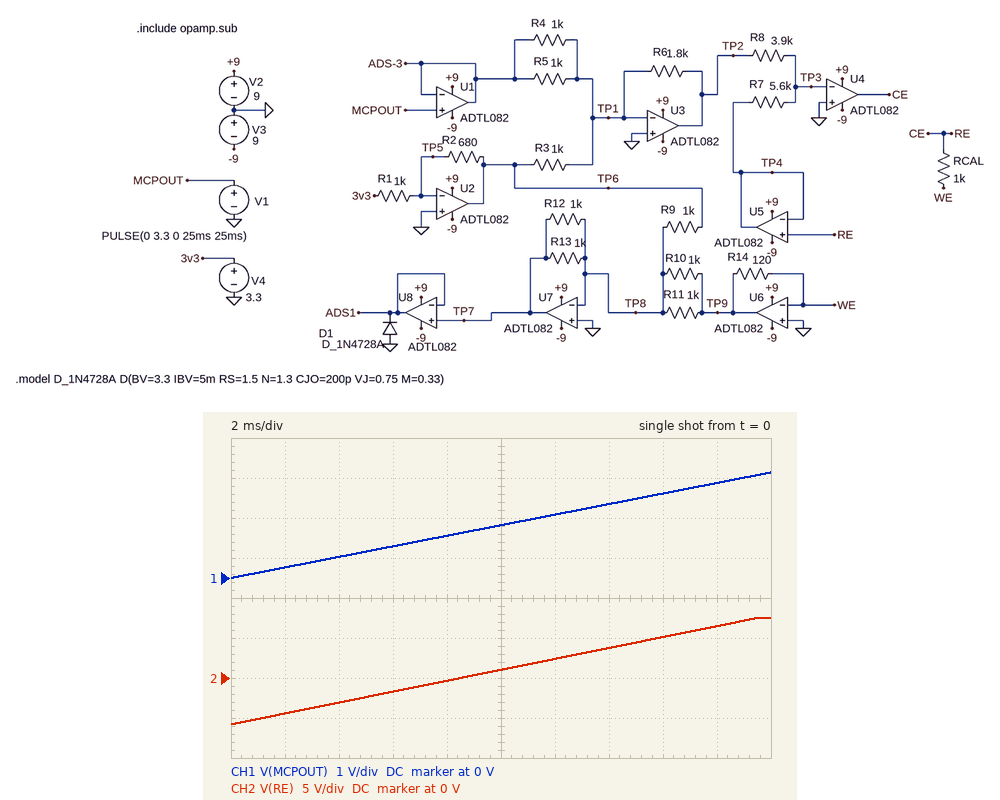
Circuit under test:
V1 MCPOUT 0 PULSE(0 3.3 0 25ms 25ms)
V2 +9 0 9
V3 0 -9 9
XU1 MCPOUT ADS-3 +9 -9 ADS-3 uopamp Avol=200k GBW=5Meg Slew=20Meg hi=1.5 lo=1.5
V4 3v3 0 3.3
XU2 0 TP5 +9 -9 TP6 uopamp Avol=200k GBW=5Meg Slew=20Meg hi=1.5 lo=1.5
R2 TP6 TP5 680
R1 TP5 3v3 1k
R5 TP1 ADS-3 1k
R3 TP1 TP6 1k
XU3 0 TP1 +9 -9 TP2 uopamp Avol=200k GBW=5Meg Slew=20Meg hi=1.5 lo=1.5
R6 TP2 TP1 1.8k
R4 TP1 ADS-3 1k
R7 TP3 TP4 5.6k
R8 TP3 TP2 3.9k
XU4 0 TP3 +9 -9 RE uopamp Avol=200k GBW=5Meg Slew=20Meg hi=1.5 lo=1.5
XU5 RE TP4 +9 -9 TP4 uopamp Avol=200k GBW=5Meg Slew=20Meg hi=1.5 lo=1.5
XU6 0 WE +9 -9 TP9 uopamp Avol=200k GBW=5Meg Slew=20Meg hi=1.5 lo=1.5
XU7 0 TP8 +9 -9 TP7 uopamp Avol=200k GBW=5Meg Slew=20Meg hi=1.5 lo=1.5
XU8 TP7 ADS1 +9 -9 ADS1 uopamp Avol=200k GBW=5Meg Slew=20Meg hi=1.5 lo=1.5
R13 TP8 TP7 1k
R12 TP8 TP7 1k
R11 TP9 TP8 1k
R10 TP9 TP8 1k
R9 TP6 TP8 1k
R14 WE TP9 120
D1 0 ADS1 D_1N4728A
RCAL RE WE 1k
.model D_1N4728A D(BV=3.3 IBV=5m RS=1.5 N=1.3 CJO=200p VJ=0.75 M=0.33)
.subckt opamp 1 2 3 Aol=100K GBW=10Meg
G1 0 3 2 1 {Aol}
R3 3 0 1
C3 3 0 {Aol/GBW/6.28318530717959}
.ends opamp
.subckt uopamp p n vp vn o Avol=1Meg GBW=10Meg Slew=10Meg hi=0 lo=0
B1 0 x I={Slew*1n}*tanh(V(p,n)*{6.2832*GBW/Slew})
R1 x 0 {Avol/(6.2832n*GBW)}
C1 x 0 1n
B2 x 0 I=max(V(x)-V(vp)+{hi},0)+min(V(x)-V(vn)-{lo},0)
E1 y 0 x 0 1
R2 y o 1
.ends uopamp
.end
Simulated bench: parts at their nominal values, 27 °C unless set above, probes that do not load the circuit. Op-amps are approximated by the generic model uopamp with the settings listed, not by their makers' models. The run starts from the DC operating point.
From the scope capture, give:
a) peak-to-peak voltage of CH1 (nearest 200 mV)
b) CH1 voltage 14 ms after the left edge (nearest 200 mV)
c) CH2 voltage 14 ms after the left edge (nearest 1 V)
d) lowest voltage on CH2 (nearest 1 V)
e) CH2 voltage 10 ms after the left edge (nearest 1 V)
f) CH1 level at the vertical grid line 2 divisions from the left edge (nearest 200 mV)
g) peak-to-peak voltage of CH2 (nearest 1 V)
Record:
2.6 V
1.8 V
4 V
-6 V
1 V
600 mV
13 V
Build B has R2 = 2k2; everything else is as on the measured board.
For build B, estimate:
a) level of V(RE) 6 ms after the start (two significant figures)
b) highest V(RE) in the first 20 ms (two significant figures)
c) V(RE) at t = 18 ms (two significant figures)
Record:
-7.5 V
-5.1 V
-6.5 V
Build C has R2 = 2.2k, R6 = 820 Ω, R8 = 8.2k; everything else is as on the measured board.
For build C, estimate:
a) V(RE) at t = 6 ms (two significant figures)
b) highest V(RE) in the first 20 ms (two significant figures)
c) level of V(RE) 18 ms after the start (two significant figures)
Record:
-3.2 V
-1.1 V
-1.4 V
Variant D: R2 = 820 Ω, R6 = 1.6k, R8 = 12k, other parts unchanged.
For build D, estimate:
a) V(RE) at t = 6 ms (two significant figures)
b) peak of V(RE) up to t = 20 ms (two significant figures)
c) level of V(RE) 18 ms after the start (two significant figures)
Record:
-840 mV
1.9 V
1.5 V
